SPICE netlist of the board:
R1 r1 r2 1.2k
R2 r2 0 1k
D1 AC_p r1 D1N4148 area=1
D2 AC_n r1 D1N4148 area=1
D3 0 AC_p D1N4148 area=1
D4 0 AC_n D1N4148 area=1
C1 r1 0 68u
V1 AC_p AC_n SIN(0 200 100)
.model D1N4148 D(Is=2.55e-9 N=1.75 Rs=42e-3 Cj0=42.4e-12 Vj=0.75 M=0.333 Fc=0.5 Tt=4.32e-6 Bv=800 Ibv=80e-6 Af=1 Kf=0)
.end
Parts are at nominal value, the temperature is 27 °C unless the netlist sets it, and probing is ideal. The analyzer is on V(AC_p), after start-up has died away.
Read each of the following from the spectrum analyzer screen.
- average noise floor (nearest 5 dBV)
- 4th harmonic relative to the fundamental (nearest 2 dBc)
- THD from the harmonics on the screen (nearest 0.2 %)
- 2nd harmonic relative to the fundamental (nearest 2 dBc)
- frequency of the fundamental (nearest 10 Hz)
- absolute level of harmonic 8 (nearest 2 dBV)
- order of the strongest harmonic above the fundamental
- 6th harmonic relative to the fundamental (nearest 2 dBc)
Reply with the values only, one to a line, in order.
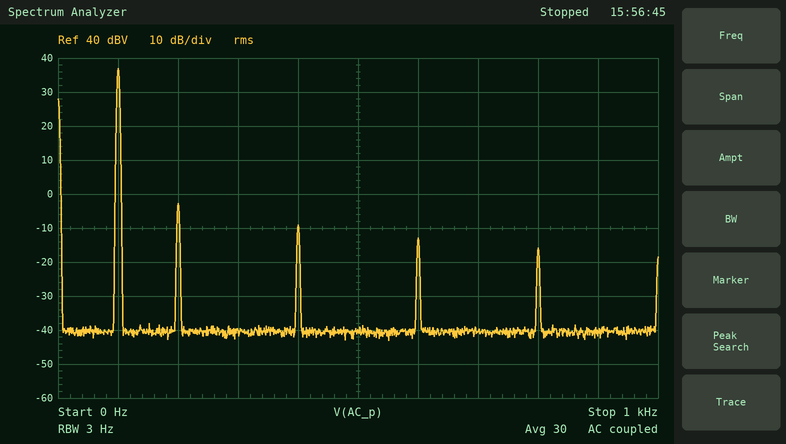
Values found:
-40 dBV
-46 dBc
1.2 %
-40 dBc
100 Hz
-16 dBV
2
-50 dBc
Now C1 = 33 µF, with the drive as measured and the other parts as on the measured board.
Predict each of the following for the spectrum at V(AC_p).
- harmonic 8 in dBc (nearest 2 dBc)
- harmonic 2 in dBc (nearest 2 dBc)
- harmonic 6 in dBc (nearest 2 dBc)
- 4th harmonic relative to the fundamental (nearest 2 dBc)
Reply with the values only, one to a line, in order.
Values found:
-48 dBc
-34 dBc
-44 dBc
-40 dBc
